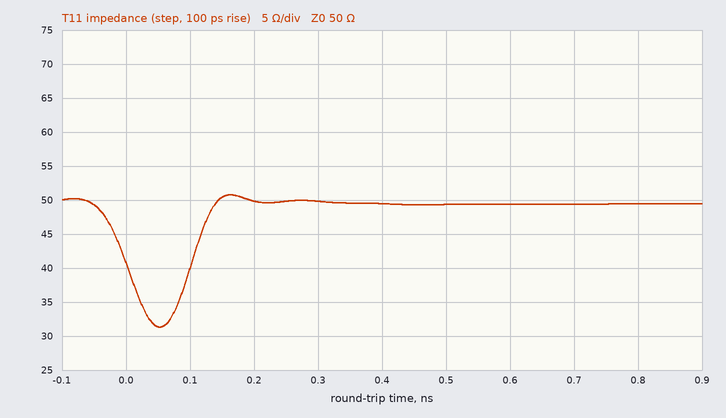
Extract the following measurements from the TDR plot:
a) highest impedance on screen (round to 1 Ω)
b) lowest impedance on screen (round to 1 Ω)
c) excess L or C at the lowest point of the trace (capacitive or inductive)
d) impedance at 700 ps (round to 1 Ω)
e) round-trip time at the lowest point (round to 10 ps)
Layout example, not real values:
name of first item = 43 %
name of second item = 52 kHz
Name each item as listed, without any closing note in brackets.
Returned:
highest impedance on screen = 51 Ω
lowest impedance on screen = 31 Ω
excess L or C at the lowest point of the trace = capacitive
impedance at 700 ps = 49 Ω
round-trip time at the lowest point = 50 ps
